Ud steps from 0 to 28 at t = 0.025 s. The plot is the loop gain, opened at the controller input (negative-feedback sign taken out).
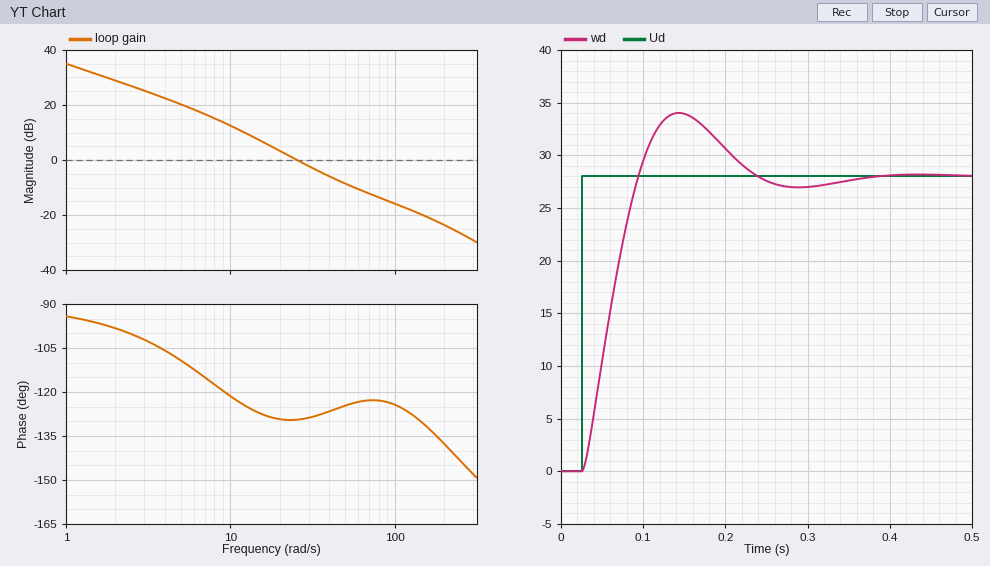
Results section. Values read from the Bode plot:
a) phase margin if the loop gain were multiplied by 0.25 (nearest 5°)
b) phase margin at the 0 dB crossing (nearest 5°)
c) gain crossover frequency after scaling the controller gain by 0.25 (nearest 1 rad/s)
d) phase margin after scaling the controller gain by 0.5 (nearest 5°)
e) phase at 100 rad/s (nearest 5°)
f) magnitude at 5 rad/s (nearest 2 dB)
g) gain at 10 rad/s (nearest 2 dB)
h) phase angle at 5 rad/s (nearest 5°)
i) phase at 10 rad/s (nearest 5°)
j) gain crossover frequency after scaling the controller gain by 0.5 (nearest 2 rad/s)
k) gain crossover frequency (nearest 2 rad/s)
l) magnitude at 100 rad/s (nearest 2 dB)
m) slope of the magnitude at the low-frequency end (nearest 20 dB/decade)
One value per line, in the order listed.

60°
50°
10 rad/s
50°
-125°
20 dB
12 dB
-110°
-120°
16 rad/s
26 rad/s
-16 dB
-20 dB/decade
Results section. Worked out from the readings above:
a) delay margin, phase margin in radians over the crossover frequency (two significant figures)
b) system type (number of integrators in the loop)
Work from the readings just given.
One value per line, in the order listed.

0.034 s
1
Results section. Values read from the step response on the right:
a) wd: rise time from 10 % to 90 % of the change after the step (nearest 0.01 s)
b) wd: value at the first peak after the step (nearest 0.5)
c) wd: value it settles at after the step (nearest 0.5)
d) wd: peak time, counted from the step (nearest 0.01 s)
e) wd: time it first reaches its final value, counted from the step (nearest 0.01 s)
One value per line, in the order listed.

0.05 s
34.0
28.0
0.12 s
0.07 s
